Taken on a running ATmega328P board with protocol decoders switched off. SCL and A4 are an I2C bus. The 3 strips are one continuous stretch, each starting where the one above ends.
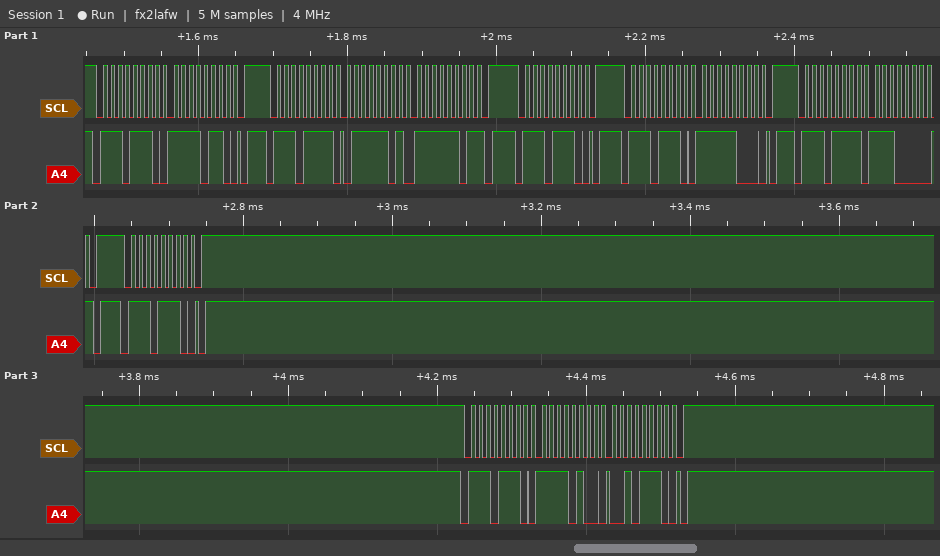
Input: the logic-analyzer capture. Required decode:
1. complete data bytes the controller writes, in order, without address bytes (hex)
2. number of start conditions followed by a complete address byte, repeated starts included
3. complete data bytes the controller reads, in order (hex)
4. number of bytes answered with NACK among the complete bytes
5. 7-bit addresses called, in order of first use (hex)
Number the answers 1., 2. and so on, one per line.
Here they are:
1. F6 F8 F4 2E
2. 7
3. 7D FD E0
4. 2
5. 0x77
